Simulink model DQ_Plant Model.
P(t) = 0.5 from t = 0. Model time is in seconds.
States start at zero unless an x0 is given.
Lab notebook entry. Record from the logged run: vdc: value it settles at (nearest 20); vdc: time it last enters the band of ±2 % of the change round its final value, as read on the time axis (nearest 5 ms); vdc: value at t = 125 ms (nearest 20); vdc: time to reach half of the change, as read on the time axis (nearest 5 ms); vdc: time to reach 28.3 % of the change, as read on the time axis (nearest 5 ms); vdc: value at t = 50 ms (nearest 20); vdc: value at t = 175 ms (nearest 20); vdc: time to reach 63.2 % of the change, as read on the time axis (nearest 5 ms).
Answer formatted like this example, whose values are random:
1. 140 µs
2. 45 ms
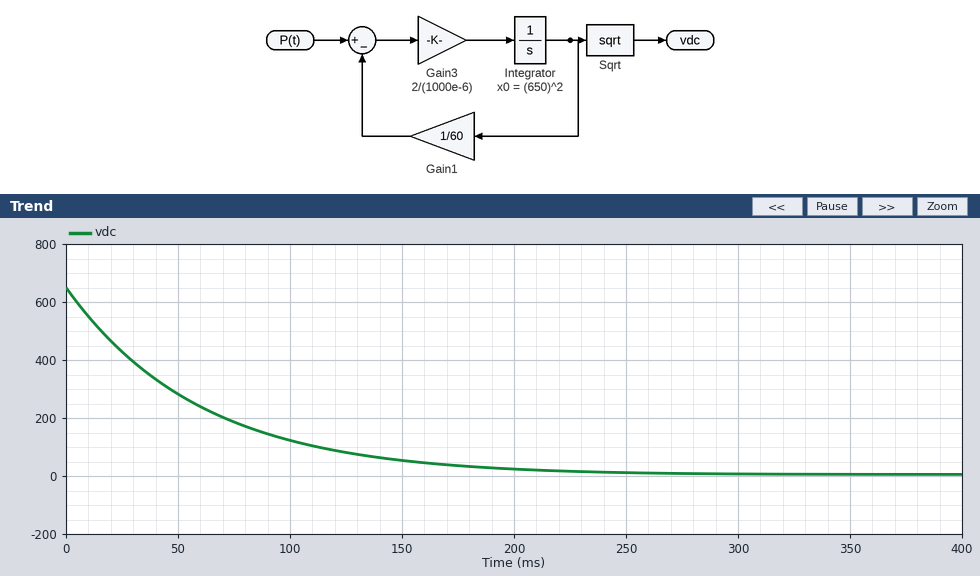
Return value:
1. 0
2. 215 ms
3. 80
4. 40 ms
5. 20 ms
6. 280
7. 40
8. 60 ms
